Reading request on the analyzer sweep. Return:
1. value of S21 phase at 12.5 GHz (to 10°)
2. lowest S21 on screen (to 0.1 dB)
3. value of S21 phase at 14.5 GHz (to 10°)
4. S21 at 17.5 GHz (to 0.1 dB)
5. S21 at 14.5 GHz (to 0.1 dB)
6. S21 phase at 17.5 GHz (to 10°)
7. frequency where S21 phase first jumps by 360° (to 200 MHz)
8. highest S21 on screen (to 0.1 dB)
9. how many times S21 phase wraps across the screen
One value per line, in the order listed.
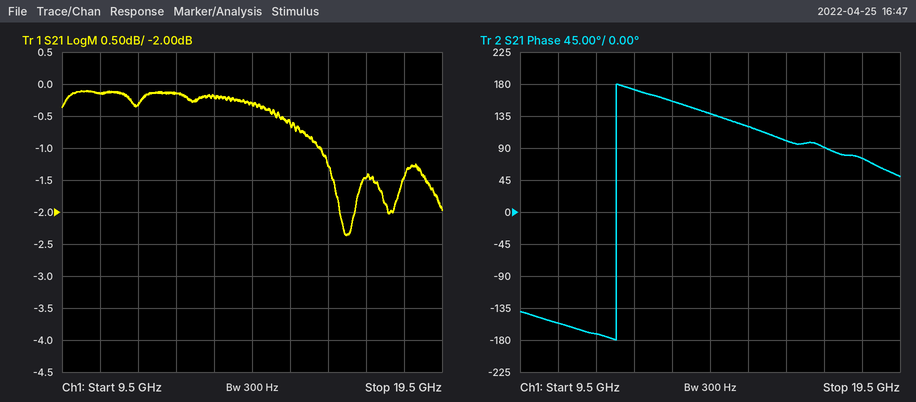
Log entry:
170°
-2.4 dB
140°
-1.5 dB
-0.3 dB
90°
12.0 GHz
-0.1 dB
1
